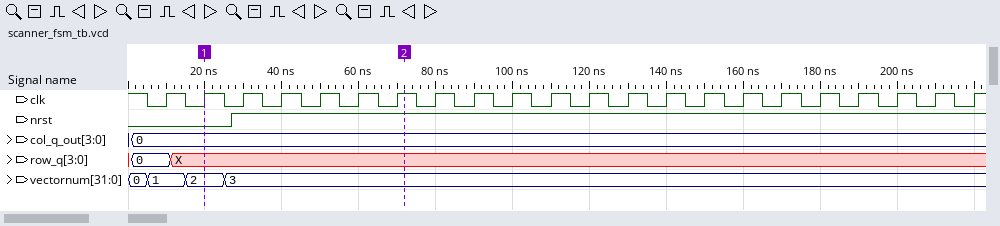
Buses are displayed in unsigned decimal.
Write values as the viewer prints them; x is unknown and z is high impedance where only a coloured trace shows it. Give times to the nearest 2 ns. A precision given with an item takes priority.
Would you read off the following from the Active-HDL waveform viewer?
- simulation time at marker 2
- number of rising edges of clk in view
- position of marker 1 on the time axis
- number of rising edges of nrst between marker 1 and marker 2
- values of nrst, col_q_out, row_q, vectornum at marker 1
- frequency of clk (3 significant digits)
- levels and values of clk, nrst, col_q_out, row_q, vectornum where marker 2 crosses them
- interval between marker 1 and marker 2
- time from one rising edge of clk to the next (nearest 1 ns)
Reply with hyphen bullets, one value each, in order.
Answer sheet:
- 72 ns
- 22
- 20 ns
- 1
- nrst=0, col_q_out=0, row_q=X, vectornum=2
- 100 MHz
- clk=1, nrst=1, col_q_out=0, row_q=X, vectornum=3
- 52 ns
- 10 ns
